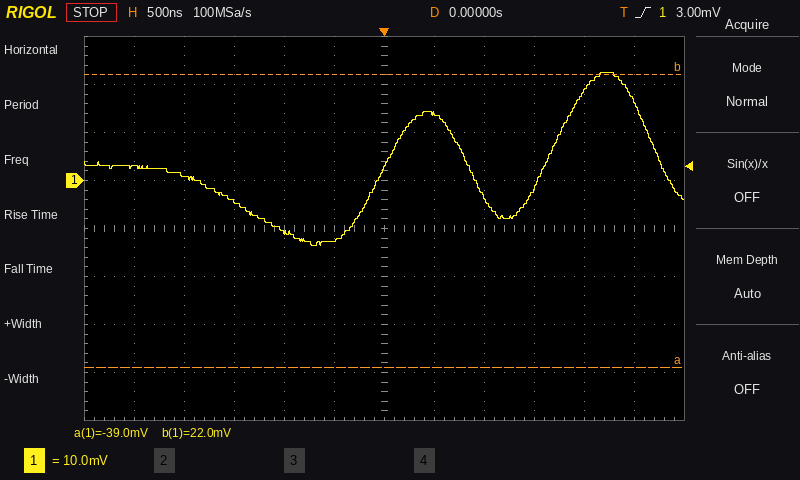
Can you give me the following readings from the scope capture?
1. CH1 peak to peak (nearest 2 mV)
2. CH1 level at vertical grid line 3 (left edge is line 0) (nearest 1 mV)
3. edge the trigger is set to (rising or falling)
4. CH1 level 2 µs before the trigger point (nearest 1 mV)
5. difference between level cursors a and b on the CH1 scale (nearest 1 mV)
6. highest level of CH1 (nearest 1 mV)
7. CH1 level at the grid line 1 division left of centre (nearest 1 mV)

36 mV
-4 mV
rising
1 mV
61 mV
22 mV
-12 mV
